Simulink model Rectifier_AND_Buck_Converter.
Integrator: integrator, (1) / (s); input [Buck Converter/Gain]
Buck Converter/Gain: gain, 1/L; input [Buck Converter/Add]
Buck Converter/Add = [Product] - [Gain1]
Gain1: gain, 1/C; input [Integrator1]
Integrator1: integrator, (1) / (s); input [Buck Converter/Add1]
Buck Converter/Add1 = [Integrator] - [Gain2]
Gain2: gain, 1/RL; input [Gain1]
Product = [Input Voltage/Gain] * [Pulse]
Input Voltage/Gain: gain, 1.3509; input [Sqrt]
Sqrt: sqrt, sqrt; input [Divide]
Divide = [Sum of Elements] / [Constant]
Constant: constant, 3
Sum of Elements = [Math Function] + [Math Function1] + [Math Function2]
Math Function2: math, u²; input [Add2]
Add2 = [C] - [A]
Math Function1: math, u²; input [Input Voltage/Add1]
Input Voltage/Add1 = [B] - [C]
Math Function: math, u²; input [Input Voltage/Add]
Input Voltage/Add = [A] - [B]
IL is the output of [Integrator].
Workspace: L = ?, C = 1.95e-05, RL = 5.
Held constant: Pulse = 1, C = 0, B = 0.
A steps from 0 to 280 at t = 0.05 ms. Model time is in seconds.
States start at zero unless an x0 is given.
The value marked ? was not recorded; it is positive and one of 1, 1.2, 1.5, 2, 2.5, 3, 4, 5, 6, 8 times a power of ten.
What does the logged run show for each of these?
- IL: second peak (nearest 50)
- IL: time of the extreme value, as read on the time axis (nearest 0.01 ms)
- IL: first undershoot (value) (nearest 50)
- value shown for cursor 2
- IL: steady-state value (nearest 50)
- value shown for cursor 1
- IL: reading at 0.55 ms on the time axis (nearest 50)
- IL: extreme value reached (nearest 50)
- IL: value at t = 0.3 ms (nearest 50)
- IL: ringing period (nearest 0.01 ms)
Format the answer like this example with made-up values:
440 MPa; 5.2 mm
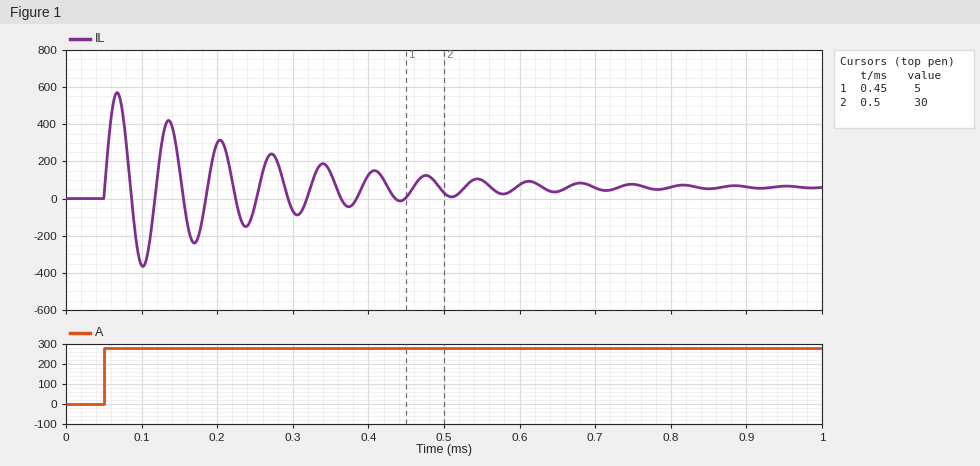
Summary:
400; 0.07 ms; -350; 30; 50; 5; 100; 550; -50; 0.07 ms
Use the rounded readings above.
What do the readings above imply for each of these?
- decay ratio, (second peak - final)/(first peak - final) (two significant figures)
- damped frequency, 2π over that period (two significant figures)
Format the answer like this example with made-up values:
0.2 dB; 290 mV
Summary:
0.70; 90 rad/ms
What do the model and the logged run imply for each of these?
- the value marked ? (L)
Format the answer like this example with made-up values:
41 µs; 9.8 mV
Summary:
6e-06
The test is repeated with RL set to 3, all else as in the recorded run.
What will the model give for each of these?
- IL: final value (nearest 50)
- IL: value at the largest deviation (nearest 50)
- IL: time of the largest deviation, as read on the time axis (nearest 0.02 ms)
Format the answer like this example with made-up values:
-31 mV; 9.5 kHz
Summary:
100; 600; 0.06 ms
